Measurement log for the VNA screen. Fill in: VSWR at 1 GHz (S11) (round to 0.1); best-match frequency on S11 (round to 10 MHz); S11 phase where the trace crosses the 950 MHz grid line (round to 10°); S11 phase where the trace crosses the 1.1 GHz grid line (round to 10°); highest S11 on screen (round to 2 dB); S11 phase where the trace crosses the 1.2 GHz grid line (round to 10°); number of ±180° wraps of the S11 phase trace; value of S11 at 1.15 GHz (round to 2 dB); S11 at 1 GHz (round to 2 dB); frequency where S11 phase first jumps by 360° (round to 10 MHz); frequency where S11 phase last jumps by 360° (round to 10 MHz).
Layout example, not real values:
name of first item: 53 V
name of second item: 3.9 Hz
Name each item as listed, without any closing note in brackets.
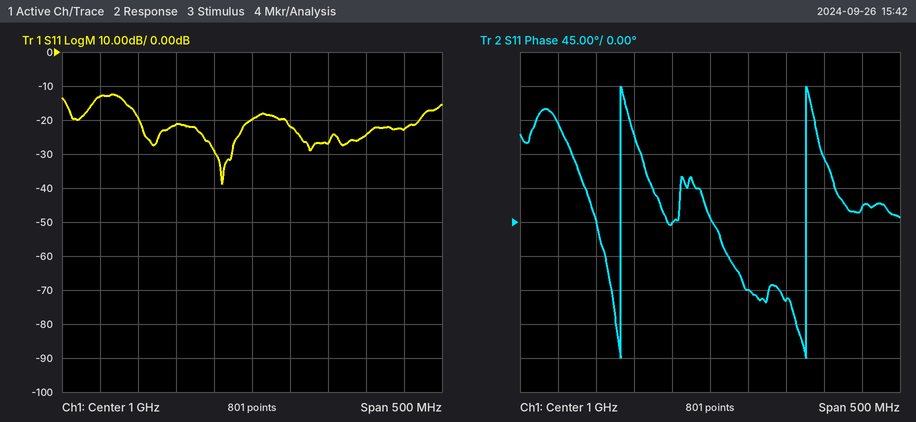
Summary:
VSWR at 1 GHz (S11): 1.2
best-match frequency on S11: 960 MHz
S11 phase where the trace crosses the 950 MHz grid line: 0°
S11 phase where the trace crosses the 1.1 GHz grid line: -100°
highest S11 on screen: -12 dB
S11 phase where the trace crosses the 1.2 GHz grid line: 20°
number of ±180° wraps of the S11 phase trace: 2
value of S11 at 1.15 GHz: -24 dB
S11 at 1 GHz: -20 dB
frequency where S11 phase first jumps by 360°: 880 MHz
frequency where S11 phase last jumps by 360°: 1.13 GHz
